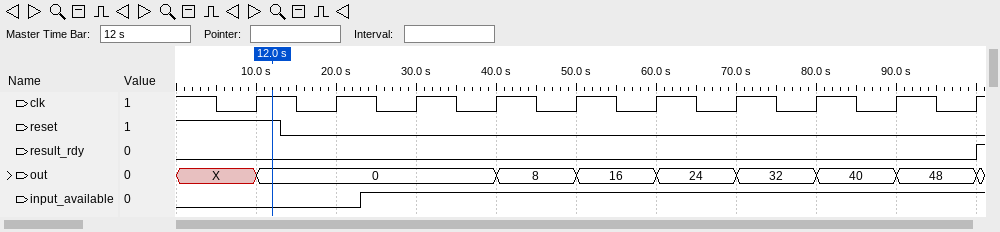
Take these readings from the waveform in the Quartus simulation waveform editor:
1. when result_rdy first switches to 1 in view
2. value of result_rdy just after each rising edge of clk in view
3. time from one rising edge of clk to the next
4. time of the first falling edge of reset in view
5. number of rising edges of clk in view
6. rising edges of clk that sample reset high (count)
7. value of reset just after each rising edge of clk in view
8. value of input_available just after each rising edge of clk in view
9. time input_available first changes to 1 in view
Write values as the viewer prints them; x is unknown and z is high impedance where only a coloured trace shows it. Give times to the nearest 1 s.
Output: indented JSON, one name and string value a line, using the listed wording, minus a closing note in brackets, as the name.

{
  "when result_rdy first switches to 1 in view": "100 s",
  "value of result_rdy just after each rising edge of clk in view": "0 0 0 0 0 0 0 0 0 1",
  "time from one rising edge of clk to the next": "10 s",
  "time of the first falling edge of reset in view": "13 s",
  "number of rising edges of clk in view": "10",
  "rising edges of clk that sample reset high": "1",
  "value of reset just after each rising edge of clk in view": "1 0 0 0 0 0 0 0 0 0",
  "value of input_available just after each rising edge of clk in view": "0 0 1 1 1 1 1 1 1 1",
  "time input_available first changes to 1 in view": "23 s"
}
